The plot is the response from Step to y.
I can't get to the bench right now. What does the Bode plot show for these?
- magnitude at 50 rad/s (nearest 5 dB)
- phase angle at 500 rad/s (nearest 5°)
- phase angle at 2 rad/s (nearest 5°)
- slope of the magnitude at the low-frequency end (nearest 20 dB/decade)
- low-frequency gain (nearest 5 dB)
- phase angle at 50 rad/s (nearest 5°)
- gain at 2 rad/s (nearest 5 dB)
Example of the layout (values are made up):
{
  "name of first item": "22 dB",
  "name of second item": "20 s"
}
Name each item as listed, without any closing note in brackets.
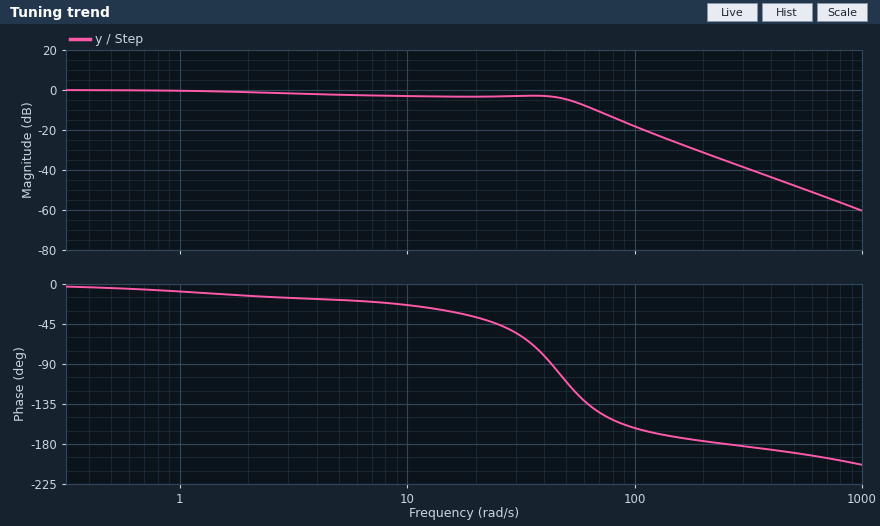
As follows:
{
  "magnitude at 50 rad/s": "-5 dB",
  "phase angle at 500 rad/s": "-190°",
  "phase angle at 2 rad/s": "-15°",
  "slope of the magnitude at the low-frequency end": "0 dB/decade",
  "low-frequency gain": "0 dB",
  "phase angle at 50 rad/s": "-110°",
  "gain at 2 rad/s": "0 dB"
}
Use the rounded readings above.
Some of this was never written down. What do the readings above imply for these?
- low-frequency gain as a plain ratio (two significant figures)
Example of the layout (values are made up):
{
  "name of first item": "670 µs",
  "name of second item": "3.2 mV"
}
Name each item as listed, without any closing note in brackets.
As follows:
{
  "low-frequency gain as a plain ratio": "1.0"
}
